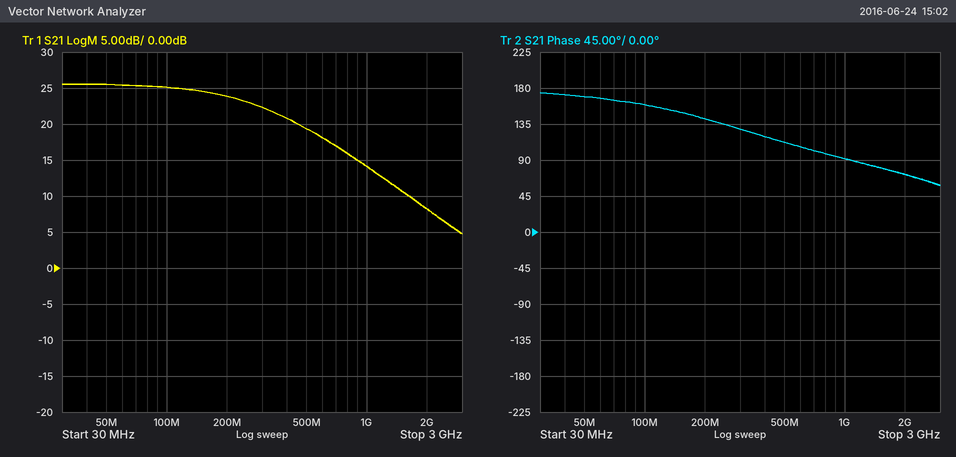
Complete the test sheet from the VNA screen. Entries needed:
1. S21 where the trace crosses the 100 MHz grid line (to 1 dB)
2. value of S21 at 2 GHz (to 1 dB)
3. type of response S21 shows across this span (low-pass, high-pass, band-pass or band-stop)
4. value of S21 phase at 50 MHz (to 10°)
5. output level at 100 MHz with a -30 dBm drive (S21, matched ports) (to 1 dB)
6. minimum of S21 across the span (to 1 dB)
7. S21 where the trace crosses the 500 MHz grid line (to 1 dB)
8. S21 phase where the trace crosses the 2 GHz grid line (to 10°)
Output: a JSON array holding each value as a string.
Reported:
["25 dB", "8 dB", "low-pass", "170°", "-5 dBm", "5 dB", "19 dB", "70°"]
